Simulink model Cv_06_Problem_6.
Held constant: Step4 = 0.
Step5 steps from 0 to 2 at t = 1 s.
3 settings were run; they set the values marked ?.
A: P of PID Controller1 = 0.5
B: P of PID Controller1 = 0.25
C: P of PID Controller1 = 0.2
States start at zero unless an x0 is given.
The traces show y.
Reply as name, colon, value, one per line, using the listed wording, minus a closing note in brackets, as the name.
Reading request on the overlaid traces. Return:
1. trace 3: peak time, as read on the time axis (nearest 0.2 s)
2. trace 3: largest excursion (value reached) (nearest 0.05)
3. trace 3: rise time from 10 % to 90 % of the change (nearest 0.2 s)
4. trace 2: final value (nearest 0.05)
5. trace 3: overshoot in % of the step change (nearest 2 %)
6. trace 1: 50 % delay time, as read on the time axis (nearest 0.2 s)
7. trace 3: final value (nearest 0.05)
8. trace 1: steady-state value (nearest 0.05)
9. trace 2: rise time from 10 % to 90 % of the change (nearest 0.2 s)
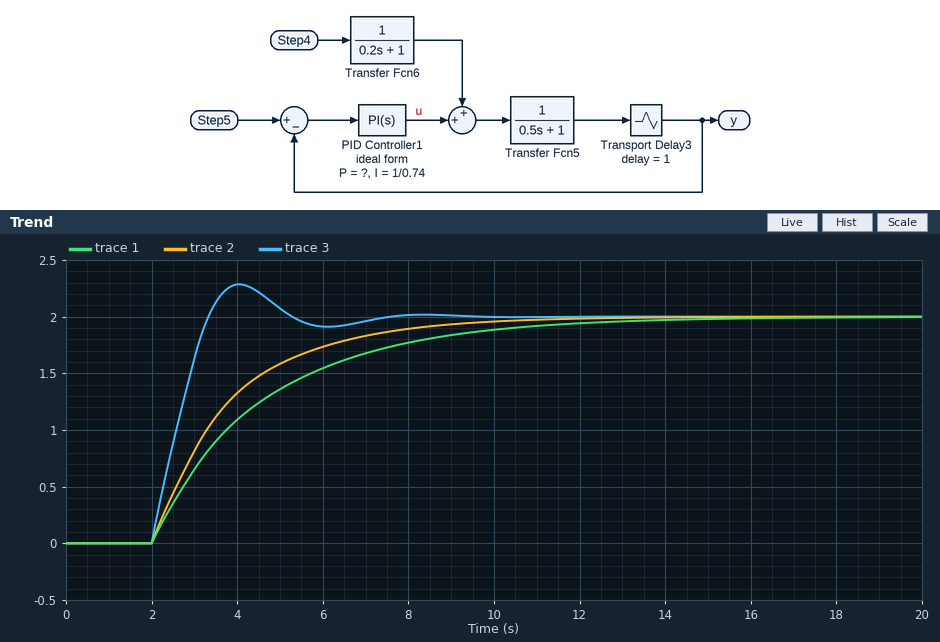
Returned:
trace 3: peak time, as read on the time axis: 4.0 s
trace 3: largest excursion (value reached): 2.30
trace 3: rise time from 10 % to 90 % of the change: 1.0 s
trace 2: final value: 2.00
trace 3: overshoot in % of the step change: 14 %
trace 1: 50 % delay time, as read on the time axis: 3.8 s
trace 3: final value: 2.00
trace 1: steady-state value: 2.00
trace 2: rise time from 10 % to 90 % of the change: 4.4 s
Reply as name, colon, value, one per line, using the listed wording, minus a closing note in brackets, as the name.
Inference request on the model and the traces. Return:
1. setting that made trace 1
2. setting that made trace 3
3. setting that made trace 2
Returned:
setting that made trace 1: C
setting that made trace 3: A
setting that made trace 2: B
